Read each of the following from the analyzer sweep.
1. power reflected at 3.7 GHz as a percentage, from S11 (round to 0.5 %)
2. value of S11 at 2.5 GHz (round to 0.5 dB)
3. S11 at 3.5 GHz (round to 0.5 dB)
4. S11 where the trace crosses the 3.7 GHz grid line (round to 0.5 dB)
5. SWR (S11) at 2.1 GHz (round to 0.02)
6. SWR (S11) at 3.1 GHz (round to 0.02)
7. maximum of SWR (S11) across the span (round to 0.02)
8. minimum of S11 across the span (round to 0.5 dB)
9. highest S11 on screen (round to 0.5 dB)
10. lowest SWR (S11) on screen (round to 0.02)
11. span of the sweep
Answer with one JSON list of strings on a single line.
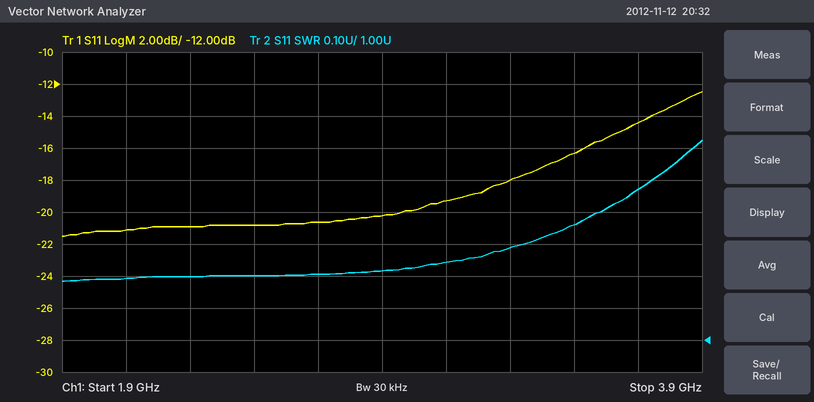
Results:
["3.5 %", "-21.0 dB", "-16.5 dB", "-14.5 dB", "1.20", "1.24", "1.62", "-21.5 dB", "-12.5 dB", "1.18", "2 GHz"]
